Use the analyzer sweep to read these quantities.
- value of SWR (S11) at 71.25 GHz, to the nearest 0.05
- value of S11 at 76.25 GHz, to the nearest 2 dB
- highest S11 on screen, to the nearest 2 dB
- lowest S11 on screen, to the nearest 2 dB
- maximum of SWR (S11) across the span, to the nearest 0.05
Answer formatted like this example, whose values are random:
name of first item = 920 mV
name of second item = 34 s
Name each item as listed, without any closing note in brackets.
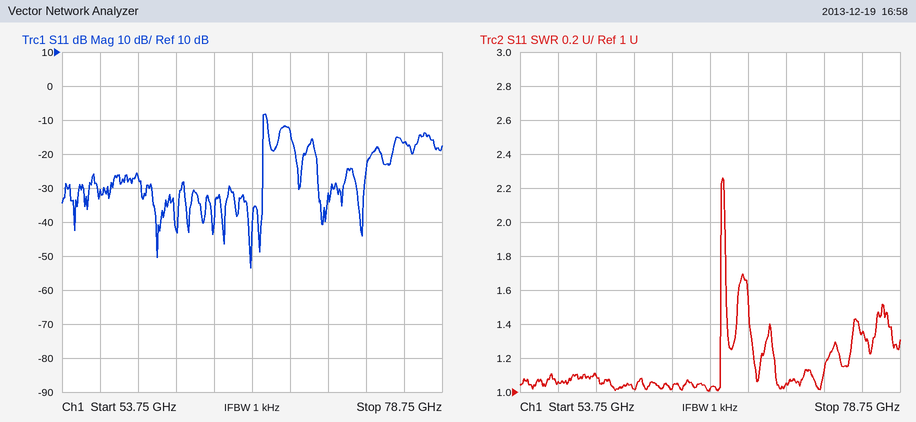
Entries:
value of SWR (S11) at 71.25 GHz, to the nearest 0.05 = 1.05
value of S11 at 76.25 GHz, to the nearest 2 dB = -16 dB
highest S11 on screen, to the nearest 2 dB = -8 dB
lowest S11 on screen, to the nearest 2 dB = -54 dB
maximum of SWR (S11) across the span, to the nearest 0.05 = 2.25
